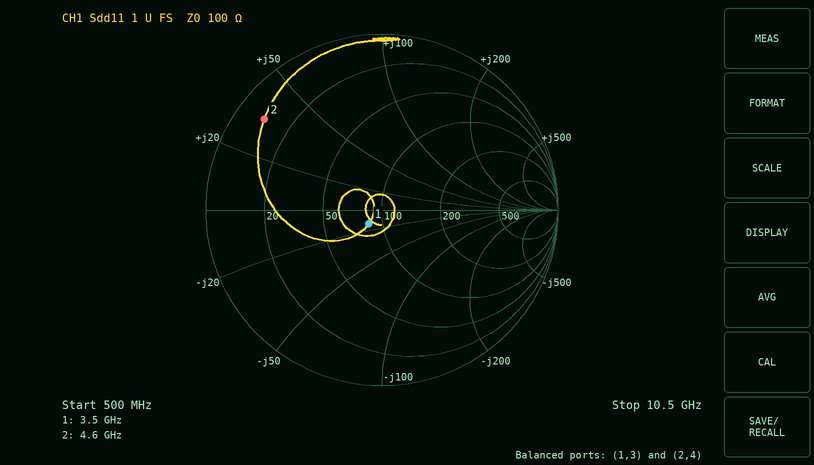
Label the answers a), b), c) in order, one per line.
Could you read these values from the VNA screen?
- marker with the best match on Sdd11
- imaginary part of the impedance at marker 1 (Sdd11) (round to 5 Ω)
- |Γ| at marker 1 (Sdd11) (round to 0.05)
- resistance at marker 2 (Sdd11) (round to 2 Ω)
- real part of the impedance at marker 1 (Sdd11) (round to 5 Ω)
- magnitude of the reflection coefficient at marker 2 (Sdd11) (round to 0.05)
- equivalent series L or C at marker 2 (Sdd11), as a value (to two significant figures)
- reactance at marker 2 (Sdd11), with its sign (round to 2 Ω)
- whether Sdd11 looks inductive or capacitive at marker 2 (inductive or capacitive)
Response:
a) marker 1
b) -15 Ω
c) 0.10
d) 10 Ω
e) 85 Ω
f) 0.85
g) 1.2 nH
h) +34 Ω
i) inductive
